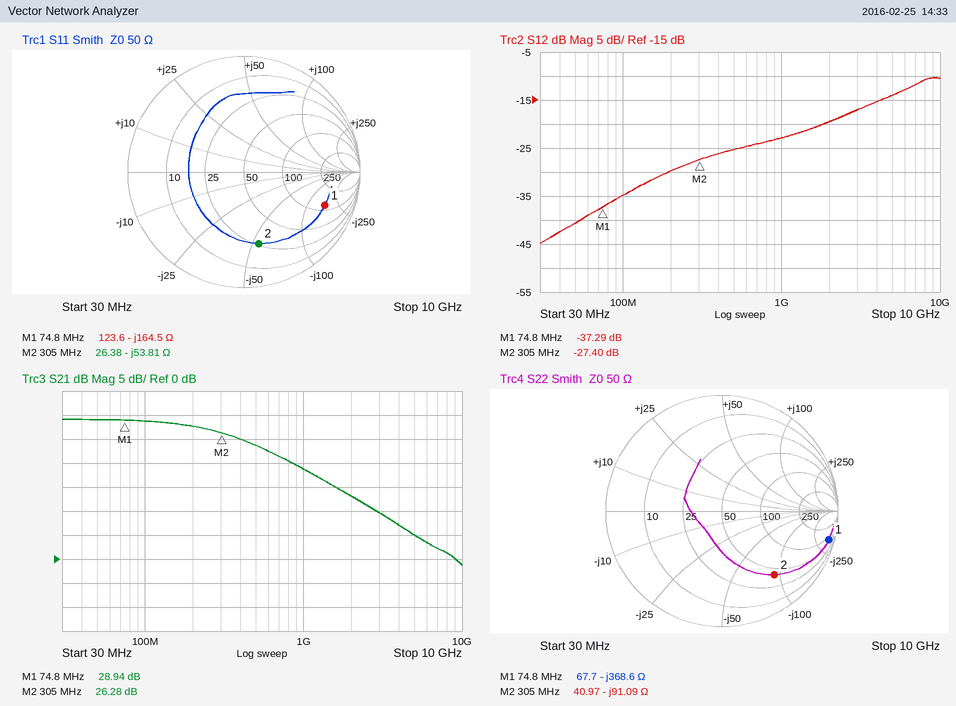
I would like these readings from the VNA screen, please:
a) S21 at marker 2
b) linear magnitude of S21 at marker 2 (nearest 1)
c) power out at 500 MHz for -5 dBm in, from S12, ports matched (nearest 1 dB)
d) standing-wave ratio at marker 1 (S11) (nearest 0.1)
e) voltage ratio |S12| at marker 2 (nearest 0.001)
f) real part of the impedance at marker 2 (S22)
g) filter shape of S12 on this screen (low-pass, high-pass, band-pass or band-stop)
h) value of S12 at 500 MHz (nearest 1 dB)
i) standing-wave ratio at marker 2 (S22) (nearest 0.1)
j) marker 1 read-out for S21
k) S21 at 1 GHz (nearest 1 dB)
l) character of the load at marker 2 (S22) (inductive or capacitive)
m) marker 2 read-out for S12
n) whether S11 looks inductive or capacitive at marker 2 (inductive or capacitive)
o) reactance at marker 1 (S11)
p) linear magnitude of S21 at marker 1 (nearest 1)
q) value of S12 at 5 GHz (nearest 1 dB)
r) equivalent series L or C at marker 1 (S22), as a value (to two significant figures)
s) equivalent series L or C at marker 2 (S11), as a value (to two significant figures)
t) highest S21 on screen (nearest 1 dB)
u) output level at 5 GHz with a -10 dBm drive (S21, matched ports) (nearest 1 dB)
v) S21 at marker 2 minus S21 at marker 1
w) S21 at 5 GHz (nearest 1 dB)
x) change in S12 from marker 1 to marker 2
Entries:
26.28 dB
21
-30 dBm
7.1
0.043
40.97 Ω
high-pass
-25 dB
5.9
28.94 dB
19 dB
capacitive
-27.40 dB
capacitive
-164.5 Ω
28
-14 dB
5.8 pF
9.7 pF
29 dB
-5 dBm
-2.66 dB
5 dB
9.89 dB
